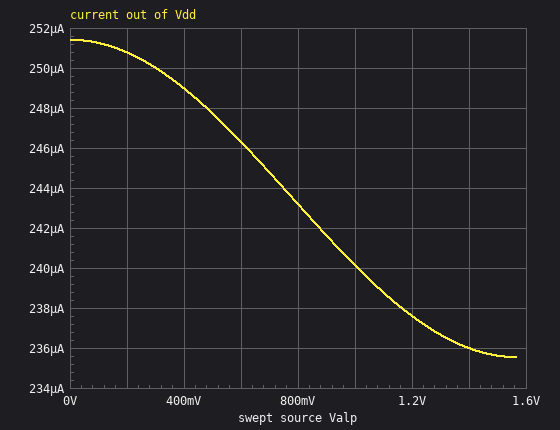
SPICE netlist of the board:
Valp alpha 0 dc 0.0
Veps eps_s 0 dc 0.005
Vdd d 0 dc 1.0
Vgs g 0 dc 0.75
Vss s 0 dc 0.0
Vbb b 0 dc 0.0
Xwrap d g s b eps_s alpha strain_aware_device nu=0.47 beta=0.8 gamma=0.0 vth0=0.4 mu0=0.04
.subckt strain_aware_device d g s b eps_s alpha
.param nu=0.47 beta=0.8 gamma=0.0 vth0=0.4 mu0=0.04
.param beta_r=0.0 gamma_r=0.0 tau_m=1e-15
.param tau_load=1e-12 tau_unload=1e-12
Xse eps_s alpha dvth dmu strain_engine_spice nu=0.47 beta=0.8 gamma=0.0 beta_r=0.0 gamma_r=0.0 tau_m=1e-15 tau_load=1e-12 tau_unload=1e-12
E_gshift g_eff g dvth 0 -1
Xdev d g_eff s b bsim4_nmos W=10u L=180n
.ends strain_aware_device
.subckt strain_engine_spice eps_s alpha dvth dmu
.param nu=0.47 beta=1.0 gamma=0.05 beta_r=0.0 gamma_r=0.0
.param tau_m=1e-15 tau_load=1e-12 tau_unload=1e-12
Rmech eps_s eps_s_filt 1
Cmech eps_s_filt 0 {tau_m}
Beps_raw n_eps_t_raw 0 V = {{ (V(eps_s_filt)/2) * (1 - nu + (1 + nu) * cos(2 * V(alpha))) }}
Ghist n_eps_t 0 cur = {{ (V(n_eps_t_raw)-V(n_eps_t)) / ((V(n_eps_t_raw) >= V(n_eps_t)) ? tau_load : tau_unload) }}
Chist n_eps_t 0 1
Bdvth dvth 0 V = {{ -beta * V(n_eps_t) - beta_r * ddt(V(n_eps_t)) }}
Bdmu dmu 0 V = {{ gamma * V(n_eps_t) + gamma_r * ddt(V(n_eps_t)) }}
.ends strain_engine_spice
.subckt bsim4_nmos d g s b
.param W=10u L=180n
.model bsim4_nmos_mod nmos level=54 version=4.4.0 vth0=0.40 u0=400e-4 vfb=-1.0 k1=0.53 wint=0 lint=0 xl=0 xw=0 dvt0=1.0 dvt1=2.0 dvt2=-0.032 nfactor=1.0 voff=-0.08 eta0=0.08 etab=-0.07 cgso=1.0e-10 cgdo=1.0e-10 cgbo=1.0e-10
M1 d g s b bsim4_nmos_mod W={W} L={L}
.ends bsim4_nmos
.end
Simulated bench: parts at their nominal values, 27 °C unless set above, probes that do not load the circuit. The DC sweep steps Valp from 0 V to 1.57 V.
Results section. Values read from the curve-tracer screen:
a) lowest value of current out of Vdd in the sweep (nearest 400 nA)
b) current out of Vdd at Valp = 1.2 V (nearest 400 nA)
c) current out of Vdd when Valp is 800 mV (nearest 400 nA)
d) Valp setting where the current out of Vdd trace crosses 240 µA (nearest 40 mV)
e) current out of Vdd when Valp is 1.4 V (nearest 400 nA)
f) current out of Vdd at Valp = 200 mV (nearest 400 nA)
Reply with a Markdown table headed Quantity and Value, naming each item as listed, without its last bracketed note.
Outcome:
| Quantity | Value |
|---|---|
| lowest value of current out of Vdd in the sweep | 235.6 µA |
| current out of Vdd at Valp = 1.2 V | 237.6 µA |
| current out of Vdd when Valp is 800 mV | 243.2 µA |
| Valp setting where the current out of Vdd trace crosses 240 µA | 1.00 V |
| current out of Vdd when Valp is 1.4 V | 236.0 µA |
| current out of Vdd at Valp = 200 mV | 250.8 µA |
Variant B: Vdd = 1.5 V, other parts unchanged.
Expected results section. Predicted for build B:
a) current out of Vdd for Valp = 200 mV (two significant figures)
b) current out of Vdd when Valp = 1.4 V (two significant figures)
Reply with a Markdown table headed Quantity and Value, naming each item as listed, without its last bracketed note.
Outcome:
| Quantity | Value |
|---|---|
| current out of Vdd for Valp = 200 mV | 290 µA |
| current out of Vdd when Valp = 1.4 V | 270 µA |
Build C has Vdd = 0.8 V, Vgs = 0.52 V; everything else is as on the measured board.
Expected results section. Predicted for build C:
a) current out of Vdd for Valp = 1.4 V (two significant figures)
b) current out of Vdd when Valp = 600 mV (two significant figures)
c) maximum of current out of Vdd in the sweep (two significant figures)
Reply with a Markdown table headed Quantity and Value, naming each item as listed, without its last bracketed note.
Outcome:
| Quantity | Value |
|---|---|
| current out of Vdd for Valp = 1.4 V | 1.3 µA |
| current out of Vdd when Valp = 600 mV | 1.5 µA |
| maximum of current out of Vdd in the sweep | 1.6 µA |
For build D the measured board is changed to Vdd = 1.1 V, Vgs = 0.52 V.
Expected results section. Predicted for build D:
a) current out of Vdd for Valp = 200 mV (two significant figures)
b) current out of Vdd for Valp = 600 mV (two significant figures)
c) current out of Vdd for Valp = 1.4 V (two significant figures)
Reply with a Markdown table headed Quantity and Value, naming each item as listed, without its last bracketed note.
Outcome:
| Quantity | Value |
|---|---|
| current out of Vdd for Valp = 200 mV | 1.9 µA |
| current out of Vdd for Valp = 600 mV | 1.8 µA |
| current out of Vdd for Valp = 1.4 V | 1.6 µA |
